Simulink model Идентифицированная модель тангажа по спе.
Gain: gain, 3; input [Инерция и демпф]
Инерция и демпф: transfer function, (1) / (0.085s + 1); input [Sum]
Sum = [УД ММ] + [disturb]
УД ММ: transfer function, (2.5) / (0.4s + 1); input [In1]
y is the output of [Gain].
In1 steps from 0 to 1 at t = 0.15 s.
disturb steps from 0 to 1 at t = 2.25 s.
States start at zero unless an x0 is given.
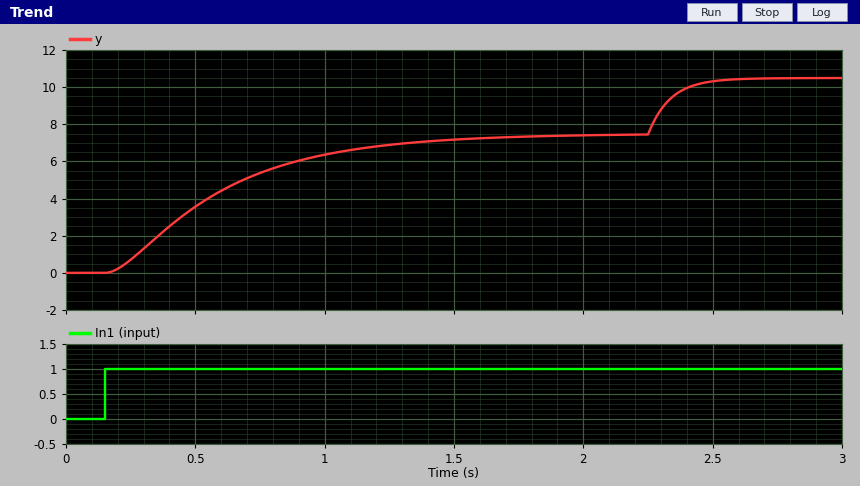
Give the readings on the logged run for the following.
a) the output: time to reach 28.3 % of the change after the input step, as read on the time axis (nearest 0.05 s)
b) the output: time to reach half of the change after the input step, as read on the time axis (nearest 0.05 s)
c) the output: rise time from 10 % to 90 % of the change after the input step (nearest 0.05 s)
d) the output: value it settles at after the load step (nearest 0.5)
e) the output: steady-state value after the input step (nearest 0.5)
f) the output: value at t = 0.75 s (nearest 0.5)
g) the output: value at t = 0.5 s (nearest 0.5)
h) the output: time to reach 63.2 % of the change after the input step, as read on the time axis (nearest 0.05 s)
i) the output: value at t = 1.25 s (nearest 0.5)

0.35 s
0.50 s
0.90 s
10.5
7.5
5.5
3.5
0.65 s
7.0
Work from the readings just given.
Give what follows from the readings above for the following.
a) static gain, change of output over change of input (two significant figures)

7.5
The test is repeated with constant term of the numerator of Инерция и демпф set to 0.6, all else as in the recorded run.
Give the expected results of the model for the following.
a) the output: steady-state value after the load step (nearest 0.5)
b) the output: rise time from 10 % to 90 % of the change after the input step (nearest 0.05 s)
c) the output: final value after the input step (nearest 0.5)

6.5
0.90 s
4.5
